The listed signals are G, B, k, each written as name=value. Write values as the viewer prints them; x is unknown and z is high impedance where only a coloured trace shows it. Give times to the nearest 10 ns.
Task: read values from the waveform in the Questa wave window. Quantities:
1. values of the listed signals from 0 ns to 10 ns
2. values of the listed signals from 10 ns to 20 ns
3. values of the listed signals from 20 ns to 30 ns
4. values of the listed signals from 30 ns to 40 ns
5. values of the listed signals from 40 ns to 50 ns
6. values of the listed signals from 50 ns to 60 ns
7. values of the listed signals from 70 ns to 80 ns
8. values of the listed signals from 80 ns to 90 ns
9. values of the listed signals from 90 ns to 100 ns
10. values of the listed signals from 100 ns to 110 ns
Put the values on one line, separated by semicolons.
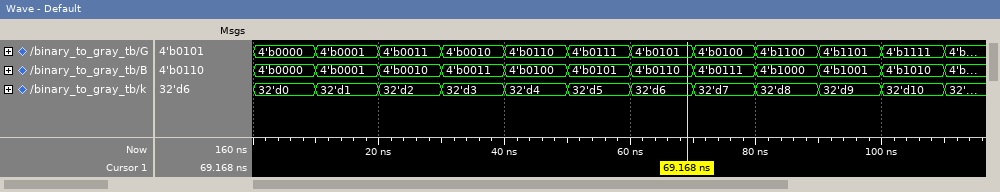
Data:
G=4'b0000, B=4'b0000, k=32'd0; G=4'b0001, B=4'b0001, k=32'd1; G=4'b0011, B=4'b0010, k=32'd2; G=4'b0010, B=4'b0011, k=32'd3; G=4'b0110, B=4'b0100, k=32'd4; G=4'b0111, B=4'b0101, k=32'd5; G=4'b0100, B=4'b0111, k=32'd7; G=4'b1100, B=4'b1000, k=32'd8; G=4'b1101, B=4'b1001, k=32'd9; G=4'b1111, B=4'b1010, k=32'd10
